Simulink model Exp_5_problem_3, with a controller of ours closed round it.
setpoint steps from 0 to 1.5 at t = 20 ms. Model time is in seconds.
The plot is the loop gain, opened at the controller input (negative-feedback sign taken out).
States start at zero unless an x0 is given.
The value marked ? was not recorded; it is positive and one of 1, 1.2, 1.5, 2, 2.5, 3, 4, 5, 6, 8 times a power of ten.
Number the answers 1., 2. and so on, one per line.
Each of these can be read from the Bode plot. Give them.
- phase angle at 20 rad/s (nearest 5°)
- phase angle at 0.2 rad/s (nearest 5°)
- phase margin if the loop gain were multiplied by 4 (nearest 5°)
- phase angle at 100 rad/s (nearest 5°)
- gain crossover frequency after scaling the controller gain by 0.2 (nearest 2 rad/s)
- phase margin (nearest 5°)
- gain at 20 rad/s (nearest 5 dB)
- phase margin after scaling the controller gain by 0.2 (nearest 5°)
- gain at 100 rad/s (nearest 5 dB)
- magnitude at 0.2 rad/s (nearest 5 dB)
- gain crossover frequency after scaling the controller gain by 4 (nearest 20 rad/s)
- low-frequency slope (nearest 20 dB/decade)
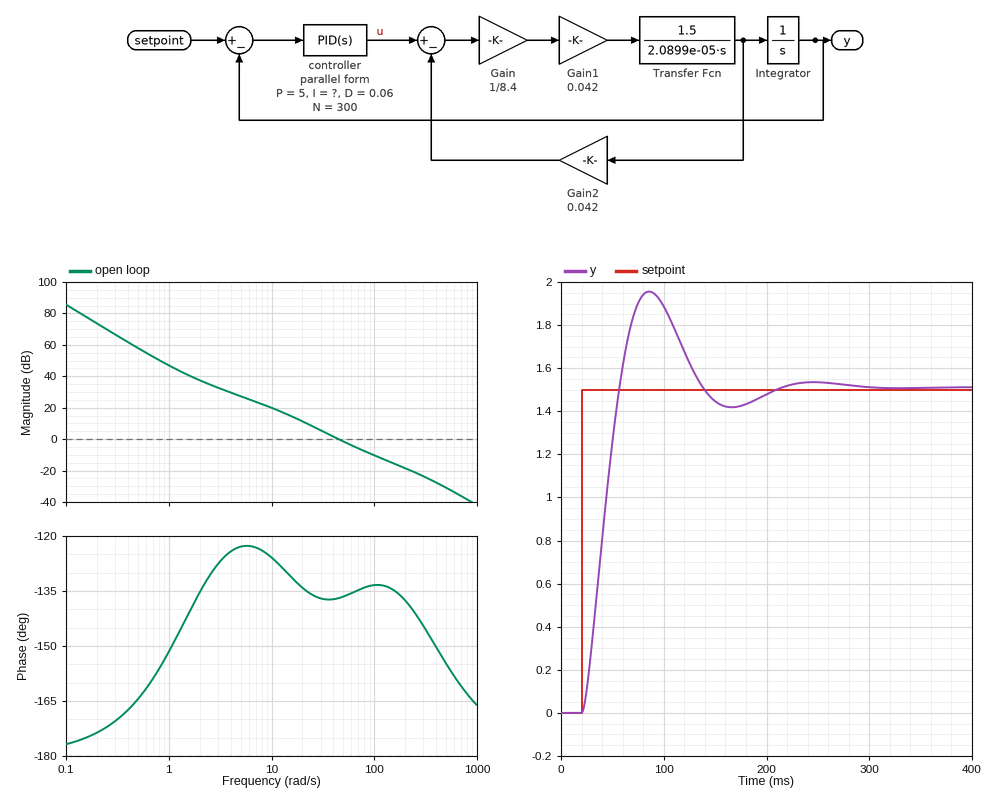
1. -135°
2. -175°
3. 45°
4. -135°
5. 16 rad/s
6. 45°
7. 10 dB
8. 50°
9. -10 dB
10. 75 dB
11. 120 rad/s
12. -40 dB/decade
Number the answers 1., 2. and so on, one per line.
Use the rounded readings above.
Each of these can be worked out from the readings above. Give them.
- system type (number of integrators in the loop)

1. 2
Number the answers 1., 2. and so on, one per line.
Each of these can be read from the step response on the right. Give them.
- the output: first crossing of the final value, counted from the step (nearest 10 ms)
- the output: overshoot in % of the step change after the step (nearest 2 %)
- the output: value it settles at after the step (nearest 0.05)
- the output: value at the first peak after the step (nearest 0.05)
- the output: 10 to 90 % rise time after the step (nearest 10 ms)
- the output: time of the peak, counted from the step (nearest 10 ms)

1. 40 ms
2. 30 %
3. 1.50
4. 1.95
5. 30 ms
6. 70 ms
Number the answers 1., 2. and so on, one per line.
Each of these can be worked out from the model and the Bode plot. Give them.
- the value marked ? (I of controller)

1. 8
